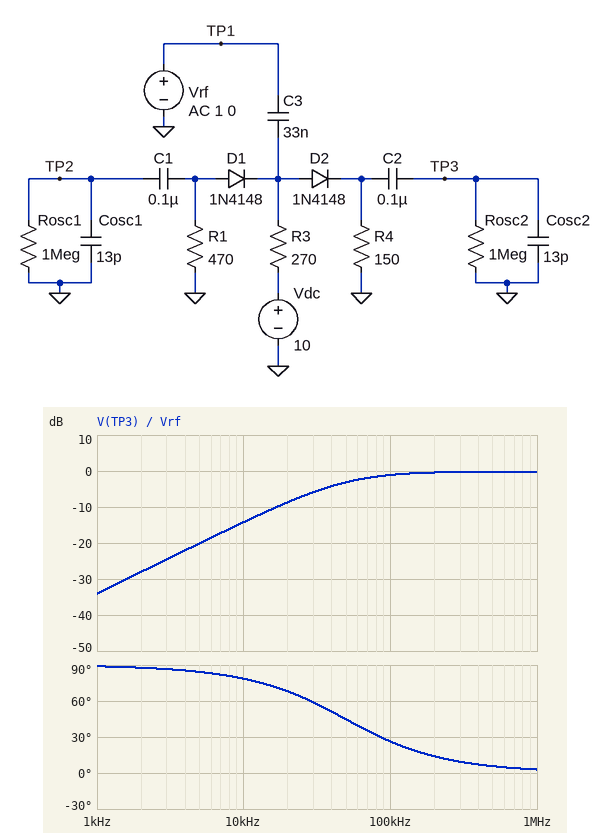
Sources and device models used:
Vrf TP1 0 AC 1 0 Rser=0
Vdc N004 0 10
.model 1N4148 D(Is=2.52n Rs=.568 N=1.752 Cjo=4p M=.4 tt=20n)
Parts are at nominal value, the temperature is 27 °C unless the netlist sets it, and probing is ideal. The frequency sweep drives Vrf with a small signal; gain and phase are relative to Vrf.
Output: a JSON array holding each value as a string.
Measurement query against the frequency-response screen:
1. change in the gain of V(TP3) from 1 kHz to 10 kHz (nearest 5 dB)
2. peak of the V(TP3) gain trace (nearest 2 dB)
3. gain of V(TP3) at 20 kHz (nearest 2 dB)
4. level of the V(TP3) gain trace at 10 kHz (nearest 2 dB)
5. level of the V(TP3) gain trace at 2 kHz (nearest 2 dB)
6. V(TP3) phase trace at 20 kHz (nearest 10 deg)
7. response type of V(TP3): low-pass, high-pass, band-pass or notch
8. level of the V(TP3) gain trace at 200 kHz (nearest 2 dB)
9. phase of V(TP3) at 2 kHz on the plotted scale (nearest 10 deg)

["20 dB", "0 dB", "-8 dB", "-14 dB", "-28 dB", "70 deg", "high-pass", "0 dB", "90 deg"]
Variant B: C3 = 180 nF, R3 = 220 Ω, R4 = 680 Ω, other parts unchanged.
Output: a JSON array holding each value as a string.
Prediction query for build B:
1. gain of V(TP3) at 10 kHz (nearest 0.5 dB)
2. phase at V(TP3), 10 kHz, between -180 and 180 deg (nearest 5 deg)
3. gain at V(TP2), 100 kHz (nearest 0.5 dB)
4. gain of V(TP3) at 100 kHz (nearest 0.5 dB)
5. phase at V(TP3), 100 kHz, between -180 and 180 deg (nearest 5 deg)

["-1.0 dB", "30 deg", "-66.0 dB", "0 dB", "5 deg"]
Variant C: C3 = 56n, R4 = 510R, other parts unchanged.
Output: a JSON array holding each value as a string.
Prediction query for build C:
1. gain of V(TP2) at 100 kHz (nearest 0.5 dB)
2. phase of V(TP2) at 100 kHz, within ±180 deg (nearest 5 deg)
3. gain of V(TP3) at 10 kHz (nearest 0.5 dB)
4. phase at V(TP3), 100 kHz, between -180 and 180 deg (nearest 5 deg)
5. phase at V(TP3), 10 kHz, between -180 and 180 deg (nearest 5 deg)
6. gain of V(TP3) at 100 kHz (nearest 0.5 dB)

["-66.0 dB", "100 deg", "-5.5 dB", "10 deg", "60 deg", "0 dB"]
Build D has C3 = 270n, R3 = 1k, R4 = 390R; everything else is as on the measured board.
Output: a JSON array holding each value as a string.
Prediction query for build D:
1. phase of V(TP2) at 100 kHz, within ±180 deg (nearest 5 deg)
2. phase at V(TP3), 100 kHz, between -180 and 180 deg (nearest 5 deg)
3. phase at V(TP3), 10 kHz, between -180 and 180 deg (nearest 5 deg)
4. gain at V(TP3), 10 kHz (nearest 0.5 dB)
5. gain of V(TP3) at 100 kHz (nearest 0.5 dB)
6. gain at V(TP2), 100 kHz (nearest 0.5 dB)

["90 deg", "0 deg", "10 deg", "-0.5 dB", "0 dB", "-63.5 dB"]
